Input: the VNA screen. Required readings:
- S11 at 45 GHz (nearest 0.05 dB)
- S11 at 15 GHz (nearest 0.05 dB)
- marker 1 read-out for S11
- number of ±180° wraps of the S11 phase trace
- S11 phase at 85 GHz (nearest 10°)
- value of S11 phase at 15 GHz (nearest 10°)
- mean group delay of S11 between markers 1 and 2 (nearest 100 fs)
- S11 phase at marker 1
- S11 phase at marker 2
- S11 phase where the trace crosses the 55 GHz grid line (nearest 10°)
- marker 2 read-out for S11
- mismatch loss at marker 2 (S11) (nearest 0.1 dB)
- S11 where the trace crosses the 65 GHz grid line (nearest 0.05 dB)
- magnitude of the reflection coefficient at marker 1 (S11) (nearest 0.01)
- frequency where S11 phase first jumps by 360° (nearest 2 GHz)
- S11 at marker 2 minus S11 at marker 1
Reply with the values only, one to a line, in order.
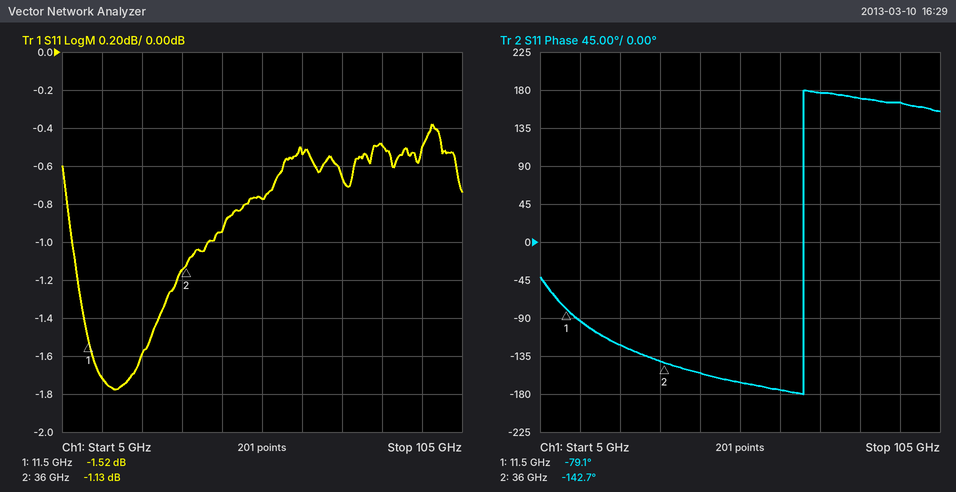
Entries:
-0.95 dB
-1.70 dB
-1.52 dB
1
170°
-90°
7.2 ps
-79.1°
-142.7°
-170°
-1.13 dB
6.4 dB
-0.55 dB
0.84
70 GHz
0.39 dB
